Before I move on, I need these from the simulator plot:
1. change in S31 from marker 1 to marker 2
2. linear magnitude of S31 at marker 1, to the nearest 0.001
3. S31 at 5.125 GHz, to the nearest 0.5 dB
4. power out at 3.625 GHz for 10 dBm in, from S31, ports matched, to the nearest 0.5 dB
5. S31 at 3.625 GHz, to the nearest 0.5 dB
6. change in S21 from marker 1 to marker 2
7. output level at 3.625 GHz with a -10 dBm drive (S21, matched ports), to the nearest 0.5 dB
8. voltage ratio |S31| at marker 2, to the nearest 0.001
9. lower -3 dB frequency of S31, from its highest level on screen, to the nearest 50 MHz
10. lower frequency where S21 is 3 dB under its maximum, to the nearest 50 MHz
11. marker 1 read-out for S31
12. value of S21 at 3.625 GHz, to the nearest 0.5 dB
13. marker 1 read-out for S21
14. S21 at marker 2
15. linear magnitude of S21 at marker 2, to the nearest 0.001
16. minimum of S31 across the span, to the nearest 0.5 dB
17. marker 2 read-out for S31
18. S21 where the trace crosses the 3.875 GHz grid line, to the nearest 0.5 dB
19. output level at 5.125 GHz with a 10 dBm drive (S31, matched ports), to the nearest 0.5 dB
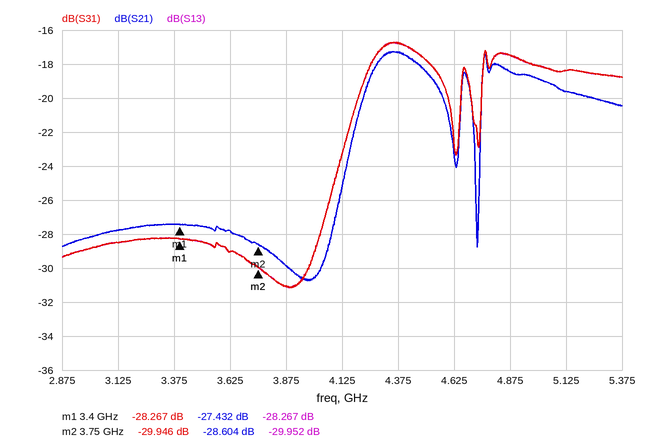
-1.679 dB
0.039
-18.5 dB
-19.0 dBm
-29.0 dB
-1.172 dB
-38.0 dBm
0.032
4.20 GHz
4.20 GHz
-28.267 dB
-28.0 dB
-27.432 dB
-28.604 dB
0.037
-31.0 dB
-29.946 dB
-30.0 dB
-8.5 dBm
